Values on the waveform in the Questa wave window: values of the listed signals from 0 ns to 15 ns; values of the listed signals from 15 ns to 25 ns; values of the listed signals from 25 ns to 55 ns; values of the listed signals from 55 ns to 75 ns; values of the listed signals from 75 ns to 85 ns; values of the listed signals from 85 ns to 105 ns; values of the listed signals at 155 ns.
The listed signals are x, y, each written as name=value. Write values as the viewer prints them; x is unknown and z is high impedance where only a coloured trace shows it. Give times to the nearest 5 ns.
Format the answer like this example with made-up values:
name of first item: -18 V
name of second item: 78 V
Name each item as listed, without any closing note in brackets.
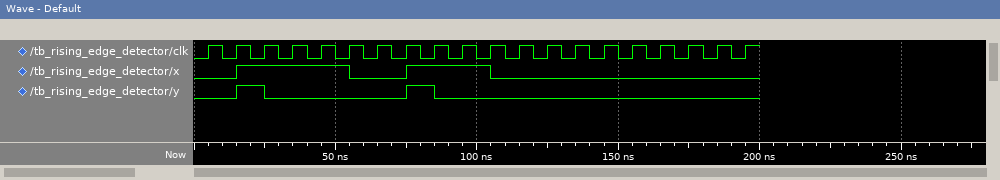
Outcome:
values of the listed signals from 0 ns to 15 ns: x=0, y=0
values of the listed signals from 15 ns to 25 ns: x=1, y=1
values of the listed signals from 25 ns to 55 ns: x=1, y=0
values of the listed signals from 55 ns to 75 ns: x=0, y=0
values of the listed signals from 75 ns to 85 ns: x=1, y=1
values of the listed signals from 85 ns to 105 ns: x=1, y=0
values of the listed signals at 155 ns: x=0, y=0
